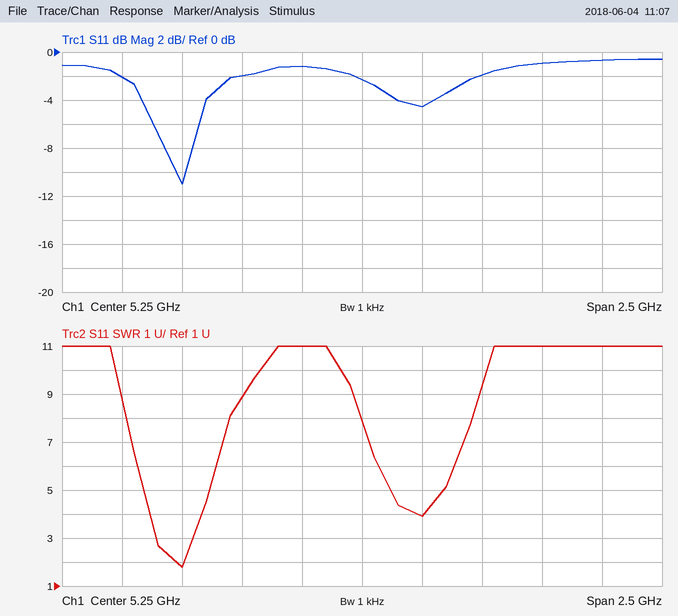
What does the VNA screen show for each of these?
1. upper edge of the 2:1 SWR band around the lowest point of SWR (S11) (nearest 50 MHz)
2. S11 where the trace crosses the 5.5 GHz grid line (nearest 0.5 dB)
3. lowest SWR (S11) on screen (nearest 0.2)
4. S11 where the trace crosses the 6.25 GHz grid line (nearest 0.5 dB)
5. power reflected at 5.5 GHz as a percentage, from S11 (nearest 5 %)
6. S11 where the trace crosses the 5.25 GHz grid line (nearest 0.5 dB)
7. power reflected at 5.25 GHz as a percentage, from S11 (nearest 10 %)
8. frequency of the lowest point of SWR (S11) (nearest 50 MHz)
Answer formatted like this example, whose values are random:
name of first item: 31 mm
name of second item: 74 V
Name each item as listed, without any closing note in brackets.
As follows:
upper edge of the 2:1 SWR band around the lowest point of SWR (S11): 4.50 GHz
S11 where the trace crosses the 5.5 GHz grid line: -4.5 dB
lowest SWR (S11) on screen: 1.8
S11 where the trace crosses the 6.25 GHz grid line: -0.5 dB
power reflected at 5.5 GHz as a percentage, from S11: 35 %
S11 where the trace crosses the 5.25 GHz grid line: -2.5 dB
power reflected at 5.25 GHz as a percentage, from S11: 60 %
frequency of the lowest point of SWR (S11): 4.50 GHz
